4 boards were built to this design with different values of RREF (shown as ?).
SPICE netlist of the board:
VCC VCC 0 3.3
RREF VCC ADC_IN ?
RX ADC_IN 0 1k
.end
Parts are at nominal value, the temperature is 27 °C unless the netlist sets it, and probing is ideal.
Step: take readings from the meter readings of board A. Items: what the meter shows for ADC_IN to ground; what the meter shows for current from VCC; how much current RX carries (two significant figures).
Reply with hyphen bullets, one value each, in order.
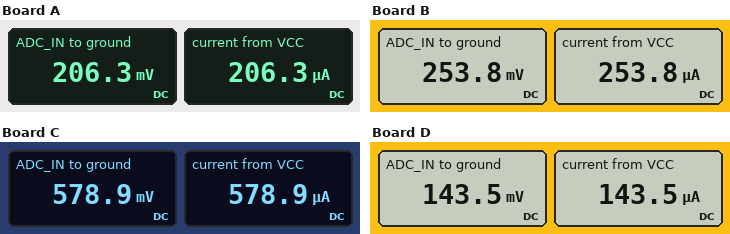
- 206.3 mV
- 206.3 µA
- 210 µA
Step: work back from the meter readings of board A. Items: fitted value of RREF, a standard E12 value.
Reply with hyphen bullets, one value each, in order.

- 15 kΩ
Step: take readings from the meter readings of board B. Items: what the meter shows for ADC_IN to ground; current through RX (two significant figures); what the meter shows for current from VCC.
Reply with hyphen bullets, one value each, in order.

- 253.8 mV
- 250 µA
- 253.8 µA
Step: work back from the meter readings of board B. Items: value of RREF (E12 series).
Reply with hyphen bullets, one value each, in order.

- 12 kΩ
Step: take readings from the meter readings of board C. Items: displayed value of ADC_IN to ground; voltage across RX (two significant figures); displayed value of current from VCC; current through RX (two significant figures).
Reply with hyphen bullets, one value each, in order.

- 578.9 mV
- 580 mV
- 578.9 µA
- 580 µA
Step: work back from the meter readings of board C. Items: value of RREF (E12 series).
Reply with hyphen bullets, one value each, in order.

- 4.7 kΩ
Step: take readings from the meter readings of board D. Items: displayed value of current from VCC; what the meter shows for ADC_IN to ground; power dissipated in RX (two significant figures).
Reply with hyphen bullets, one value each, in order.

- 143.5 µA
- 143.5 mV
- 21 µW
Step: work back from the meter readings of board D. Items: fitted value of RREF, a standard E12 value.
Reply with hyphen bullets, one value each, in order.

- 22 kΩ
